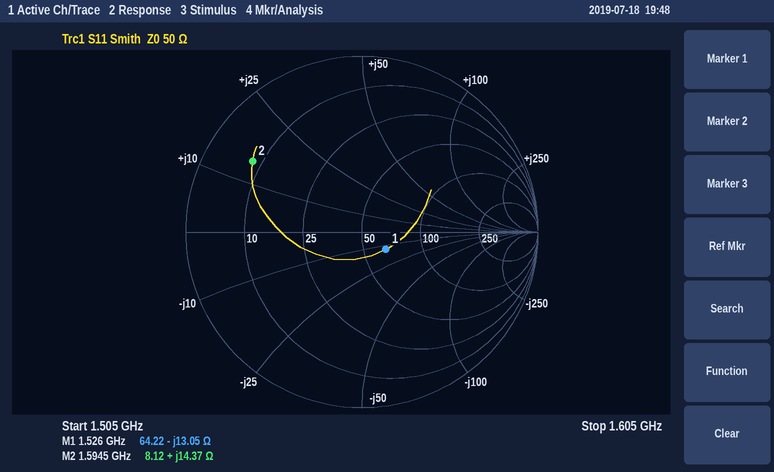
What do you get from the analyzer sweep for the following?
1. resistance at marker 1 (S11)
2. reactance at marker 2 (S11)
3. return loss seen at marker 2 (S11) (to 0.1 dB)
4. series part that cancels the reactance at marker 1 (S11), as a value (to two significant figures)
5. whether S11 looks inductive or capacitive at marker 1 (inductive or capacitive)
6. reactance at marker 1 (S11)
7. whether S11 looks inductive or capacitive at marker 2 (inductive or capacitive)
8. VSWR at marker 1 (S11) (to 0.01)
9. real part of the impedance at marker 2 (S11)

64.22 Ω
+14.37 Ω
2.6 dB
1.4 nH
capacitive
-13.05 Ω
inductive
1.40
8.12 Ω
